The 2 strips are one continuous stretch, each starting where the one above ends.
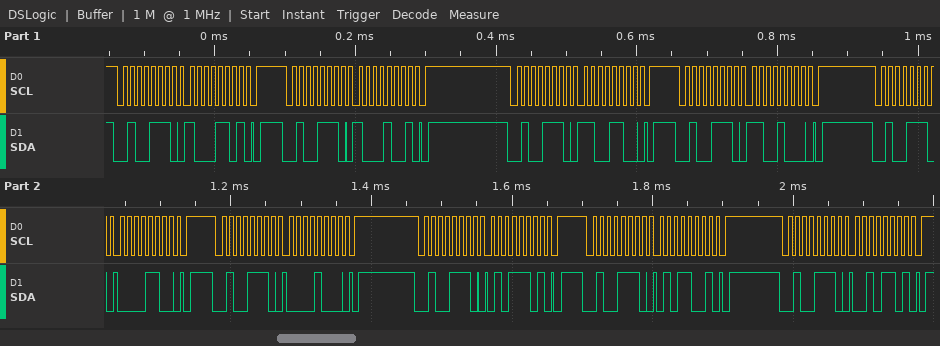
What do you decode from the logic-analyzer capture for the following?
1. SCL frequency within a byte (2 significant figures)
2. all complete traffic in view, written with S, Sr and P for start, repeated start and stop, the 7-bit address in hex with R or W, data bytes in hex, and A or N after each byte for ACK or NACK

100 kHz
S 27W A 8D A P S 27W A 89 A P S 27W A CC A P S 27W A C8 A P S 27W A 0C A P S 27W A 08 A P S 27W A 5D A P S 27W A 59 A P S 27W A 2D A P
